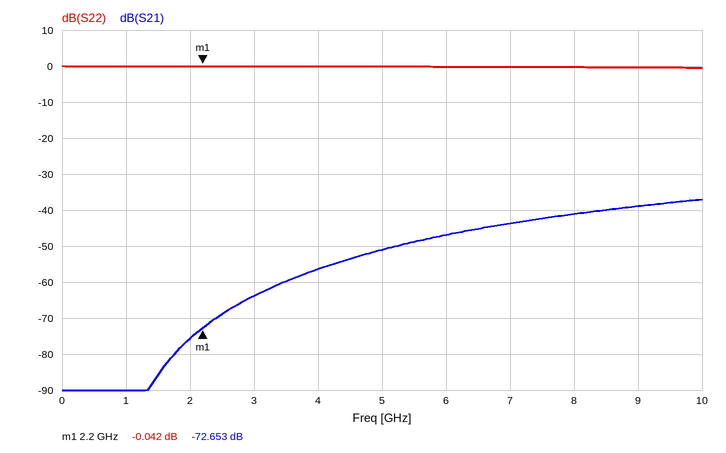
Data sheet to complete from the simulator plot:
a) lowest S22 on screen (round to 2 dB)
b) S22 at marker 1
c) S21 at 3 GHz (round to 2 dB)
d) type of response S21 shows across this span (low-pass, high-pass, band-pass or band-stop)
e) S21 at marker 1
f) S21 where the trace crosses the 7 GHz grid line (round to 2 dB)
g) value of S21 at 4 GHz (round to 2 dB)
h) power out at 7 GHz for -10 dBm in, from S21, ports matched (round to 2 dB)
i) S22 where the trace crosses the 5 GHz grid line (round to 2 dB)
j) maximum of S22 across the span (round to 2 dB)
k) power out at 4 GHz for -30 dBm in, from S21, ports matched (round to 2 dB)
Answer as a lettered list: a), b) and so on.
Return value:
a) 0 dB
b) -0.042 dB
c) -64 dB
d) high-pass
e) -72.653 dB
f) -44 dB
g) -56 dB
h) -54 dBm
i) 0 dB
j) 0 dB
k) -86 dBm
